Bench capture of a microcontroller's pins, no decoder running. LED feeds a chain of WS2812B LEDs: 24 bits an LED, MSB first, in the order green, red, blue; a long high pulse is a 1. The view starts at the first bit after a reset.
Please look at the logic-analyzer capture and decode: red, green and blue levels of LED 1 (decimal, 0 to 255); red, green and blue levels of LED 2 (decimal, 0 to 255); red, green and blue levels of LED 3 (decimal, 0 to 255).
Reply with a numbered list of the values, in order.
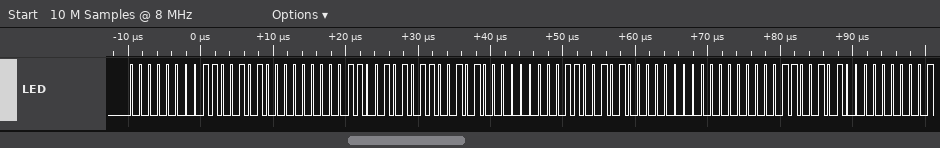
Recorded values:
1. 202, 0, 0
2. 202, 202, 0
3. 0, 202, 0
